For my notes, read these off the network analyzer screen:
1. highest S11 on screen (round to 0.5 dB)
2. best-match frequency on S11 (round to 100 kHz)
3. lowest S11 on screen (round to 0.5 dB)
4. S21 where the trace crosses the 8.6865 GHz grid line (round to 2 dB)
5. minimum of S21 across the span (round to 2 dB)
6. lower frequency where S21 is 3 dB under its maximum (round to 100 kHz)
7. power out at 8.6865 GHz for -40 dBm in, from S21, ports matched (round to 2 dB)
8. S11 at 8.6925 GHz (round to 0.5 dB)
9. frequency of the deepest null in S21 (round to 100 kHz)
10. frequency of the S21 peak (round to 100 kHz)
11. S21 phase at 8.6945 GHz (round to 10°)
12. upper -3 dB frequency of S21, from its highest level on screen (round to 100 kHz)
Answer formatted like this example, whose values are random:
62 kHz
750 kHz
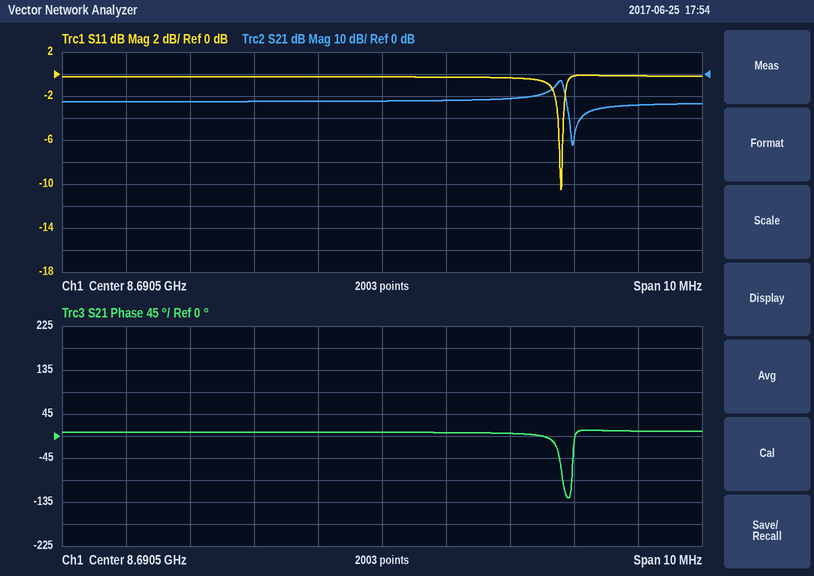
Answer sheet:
0.0 dB
8.6933 GHz
-10.5 dB
-12 dB
-32 dB
8.6932 GHz
-52 dBm
-0.5 dB
8.6935 GHz
8.6933 GHz
10°
8.6933 GHz
